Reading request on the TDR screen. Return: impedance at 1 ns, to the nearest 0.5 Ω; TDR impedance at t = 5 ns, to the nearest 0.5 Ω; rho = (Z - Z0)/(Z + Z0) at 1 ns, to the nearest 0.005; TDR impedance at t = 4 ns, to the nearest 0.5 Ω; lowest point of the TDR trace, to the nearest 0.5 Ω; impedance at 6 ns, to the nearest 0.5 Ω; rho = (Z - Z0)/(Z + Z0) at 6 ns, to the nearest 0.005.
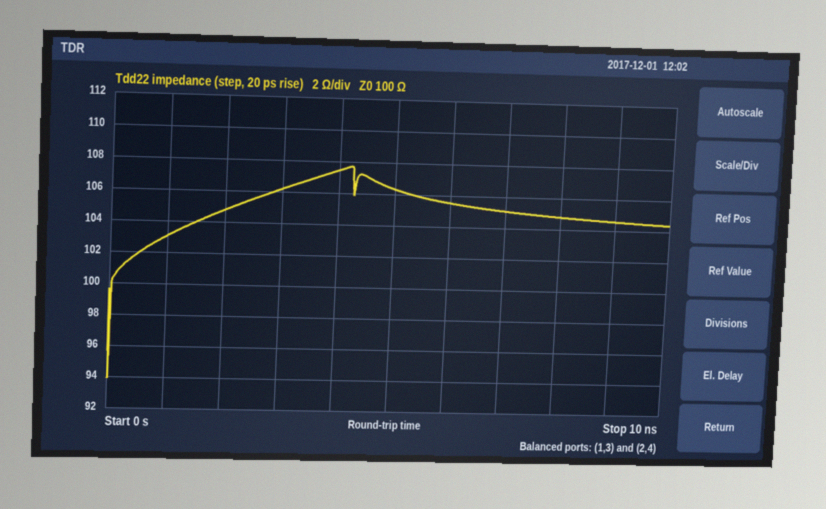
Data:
103.0 Ω
106.5 Ω
+0.015
107.5 Ω
94.0 Ω
105.5 Ω
+0.025
